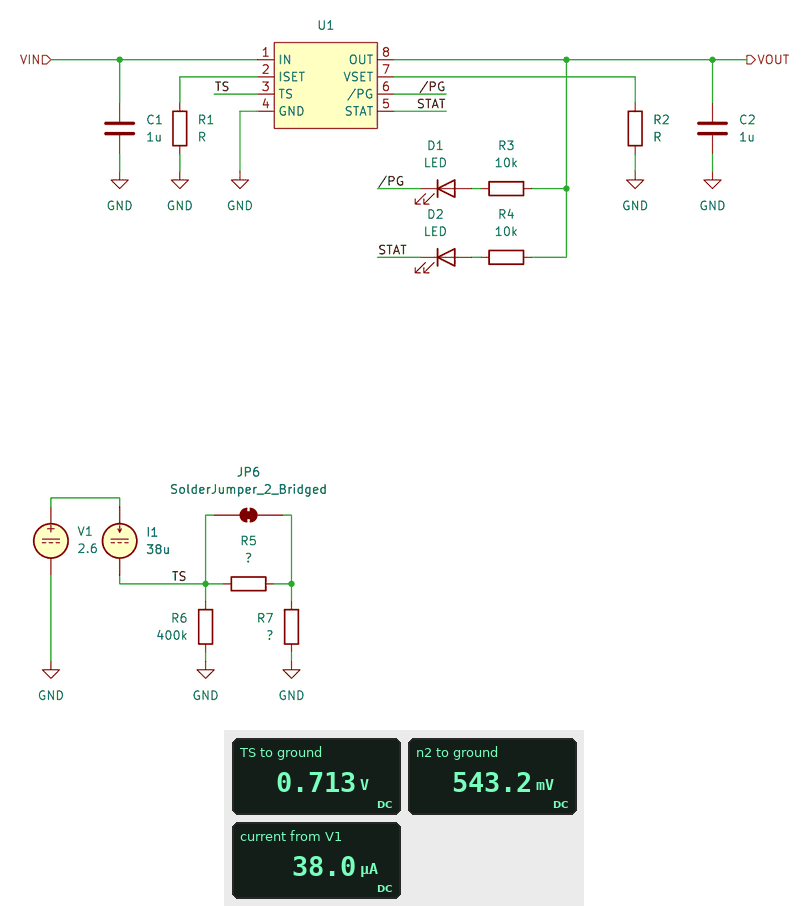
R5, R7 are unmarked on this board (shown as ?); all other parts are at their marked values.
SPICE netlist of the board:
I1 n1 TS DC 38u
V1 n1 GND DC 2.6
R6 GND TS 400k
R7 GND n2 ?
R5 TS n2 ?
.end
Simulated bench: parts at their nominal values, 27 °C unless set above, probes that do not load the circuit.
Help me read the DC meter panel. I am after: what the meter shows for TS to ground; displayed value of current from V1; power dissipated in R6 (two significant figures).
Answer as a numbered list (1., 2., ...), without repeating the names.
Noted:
1. 0.713 V
2. 38.0 µA
3. 1.3 µW
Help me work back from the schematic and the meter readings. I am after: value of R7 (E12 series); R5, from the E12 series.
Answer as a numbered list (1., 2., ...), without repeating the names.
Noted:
1. 15 kΩ
2. 4.7 kΩ
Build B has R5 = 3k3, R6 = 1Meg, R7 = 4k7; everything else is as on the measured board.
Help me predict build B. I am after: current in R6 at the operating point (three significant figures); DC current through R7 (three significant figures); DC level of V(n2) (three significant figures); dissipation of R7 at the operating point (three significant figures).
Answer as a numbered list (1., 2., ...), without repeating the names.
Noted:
1. 302 nA
2. 37.7 µA
3. 177 mV
4. 6.68 µW
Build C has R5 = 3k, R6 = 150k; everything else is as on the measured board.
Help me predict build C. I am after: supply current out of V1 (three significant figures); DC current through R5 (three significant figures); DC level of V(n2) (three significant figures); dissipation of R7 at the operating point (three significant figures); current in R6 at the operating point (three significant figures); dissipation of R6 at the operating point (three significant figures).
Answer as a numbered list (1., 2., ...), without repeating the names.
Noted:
1. 38.0 µA
2. 33.9 µA
3. 509 mV
4. 17.3 µW
5. 4.07 µA
6. 2.49 µW
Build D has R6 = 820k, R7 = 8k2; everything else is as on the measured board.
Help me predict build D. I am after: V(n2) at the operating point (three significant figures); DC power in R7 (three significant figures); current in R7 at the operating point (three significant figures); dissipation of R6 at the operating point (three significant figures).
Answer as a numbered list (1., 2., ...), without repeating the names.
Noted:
1. 307 mV
2. 11.5 µW
3. 37.4 µA
4. 284 nW
